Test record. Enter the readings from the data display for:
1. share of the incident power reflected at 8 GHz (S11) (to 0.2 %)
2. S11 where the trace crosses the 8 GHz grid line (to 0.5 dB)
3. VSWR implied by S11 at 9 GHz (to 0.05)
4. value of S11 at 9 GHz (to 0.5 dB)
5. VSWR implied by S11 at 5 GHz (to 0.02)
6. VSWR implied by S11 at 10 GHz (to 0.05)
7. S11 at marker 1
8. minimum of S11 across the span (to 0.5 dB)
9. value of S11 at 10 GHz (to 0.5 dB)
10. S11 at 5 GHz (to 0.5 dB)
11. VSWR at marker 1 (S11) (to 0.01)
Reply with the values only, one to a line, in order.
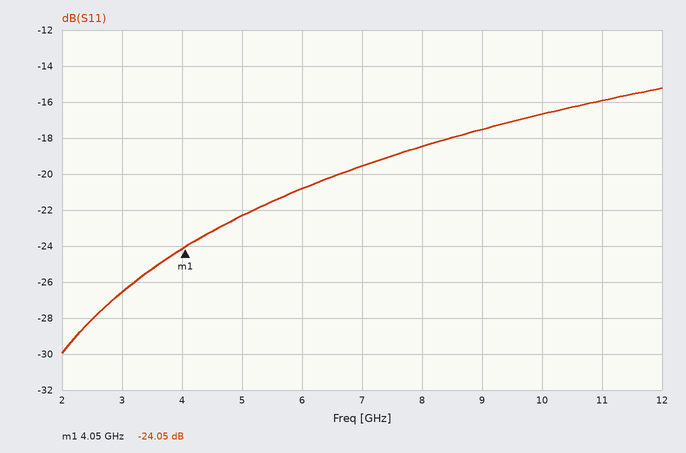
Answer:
1.4 %
-18.5 dB
1.30
-17.5 dB
1.16
1.35
-24.05 dB
-30.0 dB
-16.5 dB
-22.5 dB
1.13
